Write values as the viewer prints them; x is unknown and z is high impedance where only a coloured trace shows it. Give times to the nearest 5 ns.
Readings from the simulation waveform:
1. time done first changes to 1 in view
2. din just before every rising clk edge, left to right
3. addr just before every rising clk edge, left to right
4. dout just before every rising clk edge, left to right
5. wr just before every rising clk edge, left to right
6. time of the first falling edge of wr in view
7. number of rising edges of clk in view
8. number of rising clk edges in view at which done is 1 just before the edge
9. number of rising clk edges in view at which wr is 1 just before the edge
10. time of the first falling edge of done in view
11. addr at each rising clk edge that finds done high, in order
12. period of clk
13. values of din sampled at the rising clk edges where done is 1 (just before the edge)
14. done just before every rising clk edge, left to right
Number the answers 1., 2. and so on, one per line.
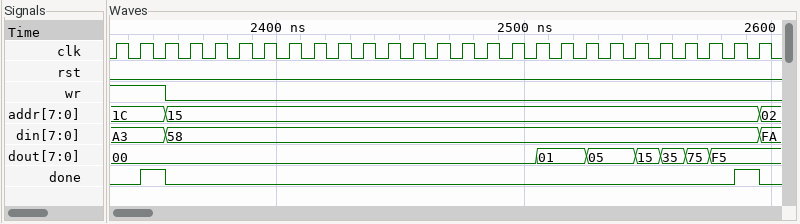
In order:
1. 2345 ns
2. A3, A3, A3, 58, 58, 58, 58, 58, 58, 58, 58, 58, 58, 58, 58, 58, 58, 58, 58, 58, 58, 58, 58, 58, 58, 58, 58
3. 1C, 1C, 1C, 15, 15, 15, 15, 15, 15, 15, 15, 15, 15, 15, 15, 15, 15, 15, 15, 15, 15, 15, 15, 15, 15, 15, 15
4. 00, 00, 00, 00, 00, 00, 00, 00, 00, 00, 00, 00, 00, 00, 00, 00, 00, 00, 01, 01, 05, 05, 15, 35, 75, F5, F5
5. 1 1 1 0 0 0 0 0 0 0 0 0 0 0 0 0 0 0 0 0 0 0 0 0 0 0 0
6. 2355 ns
7. 27
8. 2
9. 3
10. 2355 ns
11. 1C, 15
12. 10 ns
13. A3, 58
14. 0 0 1 0 0 0 0 0 0 0 0 0 0 0 0 0 0 0 0 0 0 0 0 0 0 0 1
